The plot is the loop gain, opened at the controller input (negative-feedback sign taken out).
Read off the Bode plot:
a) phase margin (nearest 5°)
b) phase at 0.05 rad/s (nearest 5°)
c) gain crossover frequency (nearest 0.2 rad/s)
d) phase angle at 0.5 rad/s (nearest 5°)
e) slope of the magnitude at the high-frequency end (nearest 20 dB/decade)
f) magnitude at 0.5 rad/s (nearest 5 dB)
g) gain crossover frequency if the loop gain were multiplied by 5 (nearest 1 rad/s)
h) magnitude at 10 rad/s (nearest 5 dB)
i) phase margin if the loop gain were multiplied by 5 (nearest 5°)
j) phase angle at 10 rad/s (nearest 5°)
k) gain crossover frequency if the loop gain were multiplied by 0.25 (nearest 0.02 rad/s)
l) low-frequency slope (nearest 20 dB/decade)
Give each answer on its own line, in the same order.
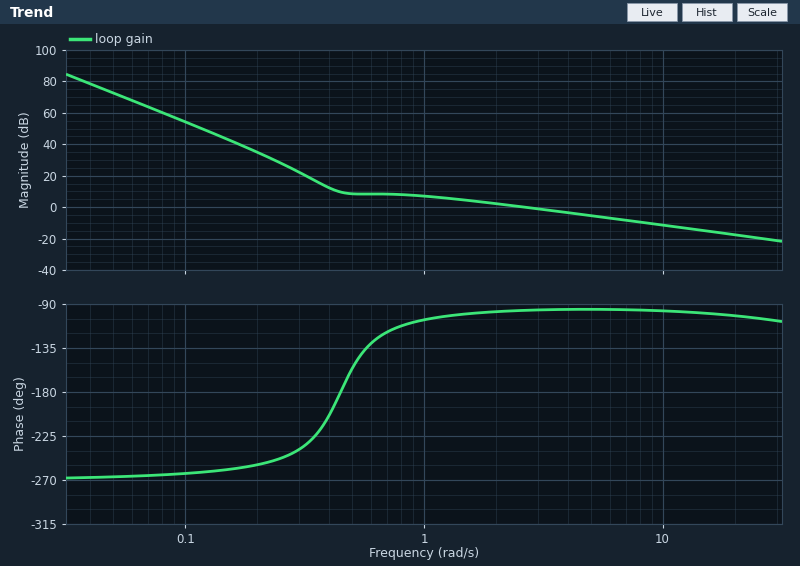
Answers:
85°
-265°
2.6 rad/s
-155°
-20 dB/decade
10 dB
13 rad/s
-10 dB
80°
-95°
0.40 rad/s
-60 dB/decade
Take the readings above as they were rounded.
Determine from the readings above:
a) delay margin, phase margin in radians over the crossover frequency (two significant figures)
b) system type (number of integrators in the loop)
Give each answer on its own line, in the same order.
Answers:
0.57 s
3
